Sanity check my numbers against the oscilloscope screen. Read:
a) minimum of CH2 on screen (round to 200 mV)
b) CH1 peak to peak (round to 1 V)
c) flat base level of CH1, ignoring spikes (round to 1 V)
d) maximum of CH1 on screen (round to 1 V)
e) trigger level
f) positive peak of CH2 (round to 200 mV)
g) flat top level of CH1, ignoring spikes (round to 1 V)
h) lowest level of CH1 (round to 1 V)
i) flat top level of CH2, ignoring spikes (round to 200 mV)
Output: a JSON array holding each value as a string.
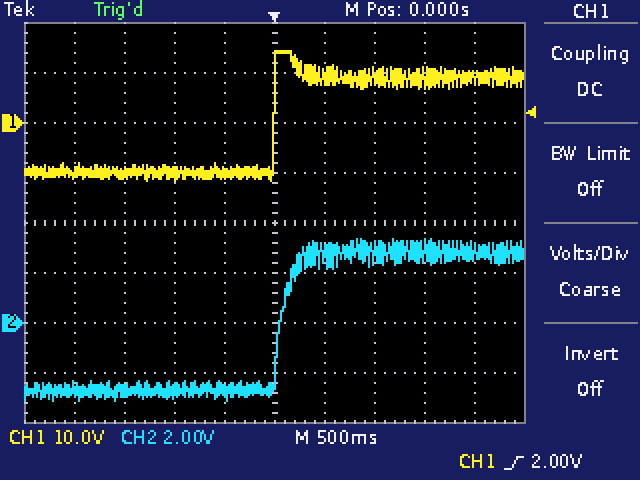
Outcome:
["-3.2 V", "26 V", "-10 V", "14 V", "2.00 V", "3.4 V", "9 V", "-12 V", "2.8 V"]
